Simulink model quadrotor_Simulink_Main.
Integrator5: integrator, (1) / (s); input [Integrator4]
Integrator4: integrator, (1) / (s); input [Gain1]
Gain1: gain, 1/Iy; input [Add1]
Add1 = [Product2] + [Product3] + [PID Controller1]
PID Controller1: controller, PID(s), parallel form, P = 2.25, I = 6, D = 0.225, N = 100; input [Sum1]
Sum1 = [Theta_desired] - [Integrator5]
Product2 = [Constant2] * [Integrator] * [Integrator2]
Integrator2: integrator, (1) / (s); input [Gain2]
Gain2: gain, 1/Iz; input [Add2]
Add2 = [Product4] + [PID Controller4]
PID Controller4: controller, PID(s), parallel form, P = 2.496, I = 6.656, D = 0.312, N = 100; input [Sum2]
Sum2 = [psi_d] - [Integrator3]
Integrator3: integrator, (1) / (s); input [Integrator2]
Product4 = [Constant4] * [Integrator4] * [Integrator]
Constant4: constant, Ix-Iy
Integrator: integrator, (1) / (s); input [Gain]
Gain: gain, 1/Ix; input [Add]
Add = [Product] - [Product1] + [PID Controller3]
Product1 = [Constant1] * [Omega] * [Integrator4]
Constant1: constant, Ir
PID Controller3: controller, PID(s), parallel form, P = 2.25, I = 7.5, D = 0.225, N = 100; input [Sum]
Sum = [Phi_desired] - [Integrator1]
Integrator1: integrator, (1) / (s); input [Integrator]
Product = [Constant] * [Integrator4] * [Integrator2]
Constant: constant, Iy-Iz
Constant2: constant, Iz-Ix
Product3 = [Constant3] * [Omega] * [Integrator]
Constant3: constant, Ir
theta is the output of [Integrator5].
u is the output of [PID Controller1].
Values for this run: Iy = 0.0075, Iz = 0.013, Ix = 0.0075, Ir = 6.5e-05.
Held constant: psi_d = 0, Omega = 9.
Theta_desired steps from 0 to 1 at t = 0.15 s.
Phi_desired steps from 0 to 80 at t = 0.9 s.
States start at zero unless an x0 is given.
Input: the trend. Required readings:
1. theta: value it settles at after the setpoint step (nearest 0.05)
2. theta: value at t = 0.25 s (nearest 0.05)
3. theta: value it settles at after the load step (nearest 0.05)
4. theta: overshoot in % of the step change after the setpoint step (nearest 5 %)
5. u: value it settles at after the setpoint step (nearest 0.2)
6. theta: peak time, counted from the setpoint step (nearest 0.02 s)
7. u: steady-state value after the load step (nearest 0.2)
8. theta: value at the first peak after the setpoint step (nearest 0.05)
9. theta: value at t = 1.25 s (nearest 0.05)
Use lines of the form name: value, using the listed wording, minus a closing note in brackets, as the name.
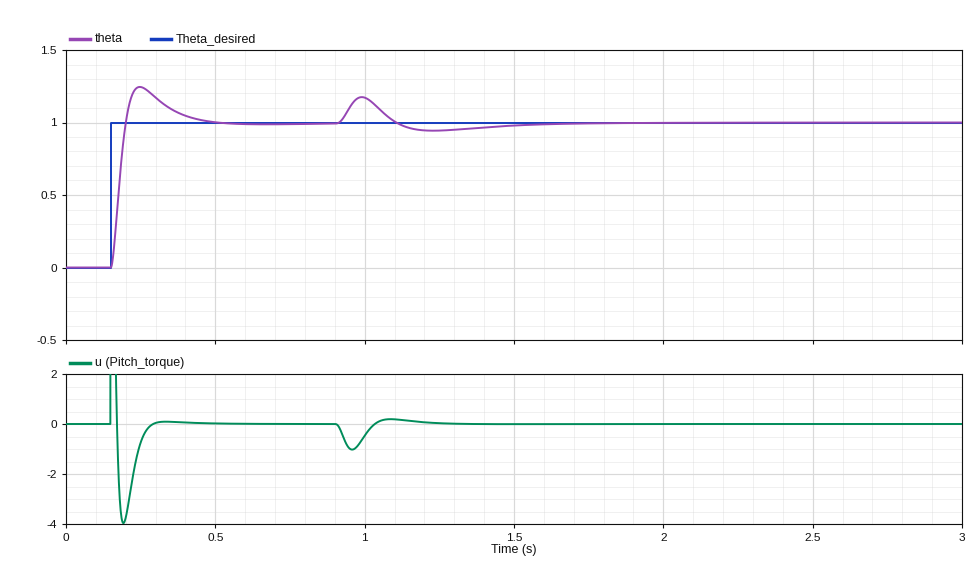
theta: value it settles at after the setpoint step: 1.00
theta: value at t = 0.25 s: 1.25
theta: value it settles at after the load step: 1.00
theta: overshoot in % of the step change after the setpoint step: 25 %
u: value it settles at after the setpoint step: 0.0
theta: peak time, counted from the setpoint step: 0.10 s
u: steady-state value after the load step: 0.0
theta: value at the first peak after the setpoint step: 1.25
theta: value at t = 1.25 s: 0.95
